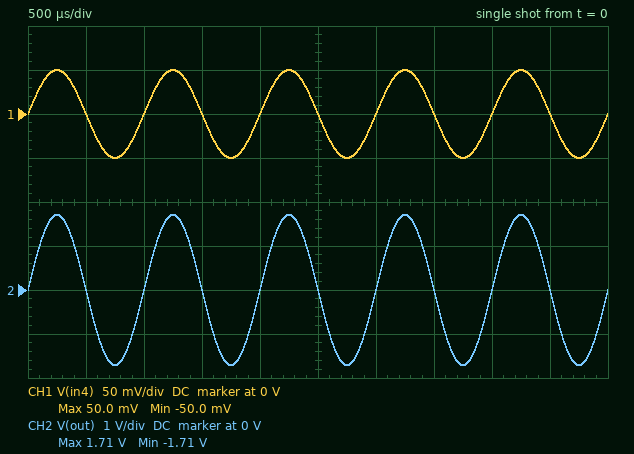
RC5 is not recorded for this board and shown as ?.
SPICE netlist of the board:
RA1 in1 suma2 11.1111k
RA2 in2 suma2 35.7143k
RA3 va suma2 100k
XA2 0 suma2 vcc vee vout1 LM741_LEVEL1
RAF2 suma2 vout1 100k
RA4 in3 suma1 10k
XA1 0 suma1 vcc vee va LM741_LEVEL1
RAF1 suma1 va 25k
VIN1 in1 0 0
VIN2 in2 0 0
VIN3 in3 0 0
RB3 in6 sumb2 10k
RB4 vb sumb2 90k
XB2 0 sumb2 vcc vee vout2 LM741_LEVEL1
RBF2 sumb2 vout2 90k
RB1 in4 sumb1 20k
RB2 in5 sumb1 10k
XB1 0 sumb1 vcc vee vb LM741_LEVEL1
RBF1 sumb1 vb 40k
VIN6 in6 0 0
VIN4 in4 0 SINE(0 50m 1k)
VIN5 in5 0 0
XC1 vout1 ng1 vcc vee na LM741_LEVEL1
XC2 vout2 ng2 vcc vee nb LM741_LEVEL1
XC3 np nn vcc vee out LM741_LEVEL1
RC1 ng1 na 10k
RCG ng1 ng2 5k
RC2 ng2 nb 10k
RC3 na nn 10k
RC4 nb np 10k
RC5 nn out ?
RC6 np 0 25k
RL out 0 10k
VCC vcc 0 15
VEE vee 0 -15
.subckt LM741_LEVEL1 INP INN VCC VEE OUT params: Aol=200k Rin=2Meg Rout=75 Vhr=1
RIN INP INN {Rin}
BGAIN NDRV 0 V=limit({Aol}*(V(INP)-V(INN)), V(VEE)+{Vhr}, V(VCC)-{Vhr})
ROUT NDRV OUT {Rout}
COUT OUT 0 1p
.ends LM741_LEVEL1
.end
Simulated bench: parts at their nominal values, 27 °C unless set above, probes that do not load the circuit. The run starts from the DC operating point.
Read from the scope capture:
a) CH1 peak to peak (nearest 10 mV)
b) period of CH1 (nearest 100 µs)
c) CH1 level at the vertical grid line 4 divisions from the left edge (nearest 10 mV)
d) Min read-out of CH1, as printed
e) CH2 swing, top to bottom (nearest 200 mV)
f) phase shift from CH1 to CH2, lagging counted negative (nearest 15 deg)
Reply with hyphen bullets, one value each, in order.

- 100 mV
- 1.0 ms
- 0 V
- -50.0 mV
- 3.4 V
- 0 deg
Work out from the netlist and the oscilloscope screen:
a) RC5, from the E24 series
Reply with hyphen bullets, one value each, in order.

- 36 kΩ
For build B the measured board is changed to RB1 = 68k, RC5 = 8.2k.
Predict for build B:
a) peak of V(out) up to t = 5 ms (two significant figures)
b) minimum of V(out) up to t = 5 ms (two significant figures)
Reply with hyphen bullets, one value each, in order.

- 160 mV
- -160 mV
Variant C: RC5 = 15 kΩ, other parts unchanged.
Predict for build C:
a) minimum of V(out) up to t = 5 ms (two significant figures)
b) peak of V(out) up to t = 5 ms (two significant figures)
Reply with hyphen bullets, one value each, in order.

- -840 mV
- 840 mV
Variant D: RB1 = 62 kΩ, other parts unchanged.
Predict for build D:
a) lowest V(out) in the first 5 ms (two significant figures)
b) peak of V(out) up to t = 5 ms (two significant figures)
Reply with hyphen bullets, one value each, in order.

- -550 mV
- 550 mV
